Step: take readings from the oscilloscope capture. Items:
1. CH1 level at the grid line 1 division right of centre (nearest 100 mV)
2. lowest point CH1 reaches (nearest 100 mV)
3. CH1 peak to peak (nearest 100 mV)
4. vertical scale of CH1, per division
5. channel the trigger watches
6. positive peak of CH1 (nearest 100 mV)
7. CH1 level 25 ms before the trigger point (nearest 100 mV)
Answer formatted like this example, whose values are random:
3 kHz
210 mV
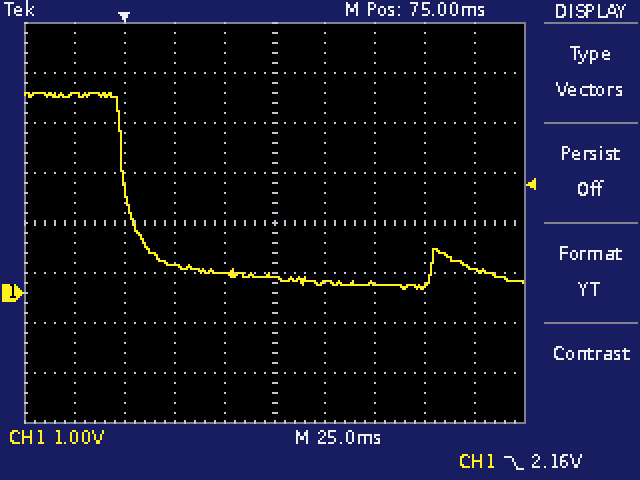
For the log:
200 mV
100 mV
3.9 V
1 V
CH1
4.0 V
4.0 V
